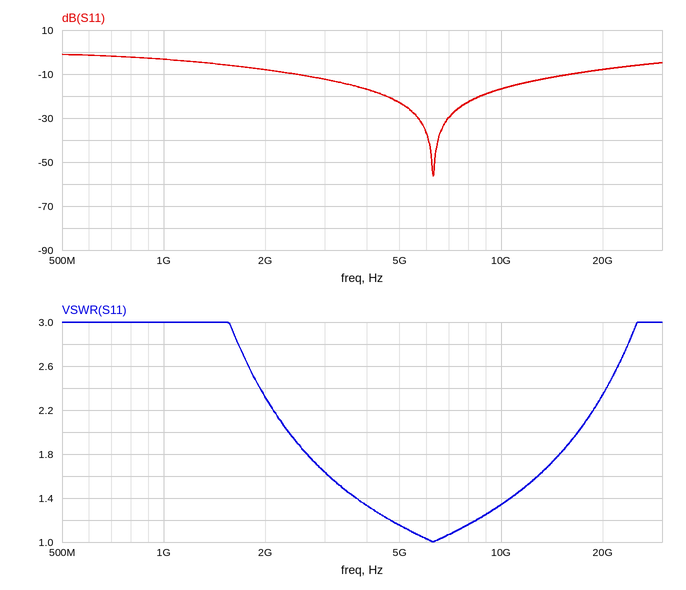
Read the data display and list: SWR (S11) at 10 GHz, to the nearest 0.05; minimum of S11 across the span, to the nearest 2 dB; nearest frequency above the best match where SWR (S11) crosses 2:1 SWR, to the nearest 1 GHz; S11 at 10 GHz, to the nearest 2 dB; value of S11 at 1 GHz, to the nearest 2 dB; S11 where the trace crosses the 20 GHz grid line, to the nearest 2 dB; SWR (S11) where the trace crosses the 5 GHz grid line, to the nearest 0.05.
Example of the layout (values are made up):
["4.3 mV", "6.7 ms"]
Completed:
["1.35", "-56 dB", "17 GHz", "-16 dB", "-4 dB", "-8 dB", "1.15"]
